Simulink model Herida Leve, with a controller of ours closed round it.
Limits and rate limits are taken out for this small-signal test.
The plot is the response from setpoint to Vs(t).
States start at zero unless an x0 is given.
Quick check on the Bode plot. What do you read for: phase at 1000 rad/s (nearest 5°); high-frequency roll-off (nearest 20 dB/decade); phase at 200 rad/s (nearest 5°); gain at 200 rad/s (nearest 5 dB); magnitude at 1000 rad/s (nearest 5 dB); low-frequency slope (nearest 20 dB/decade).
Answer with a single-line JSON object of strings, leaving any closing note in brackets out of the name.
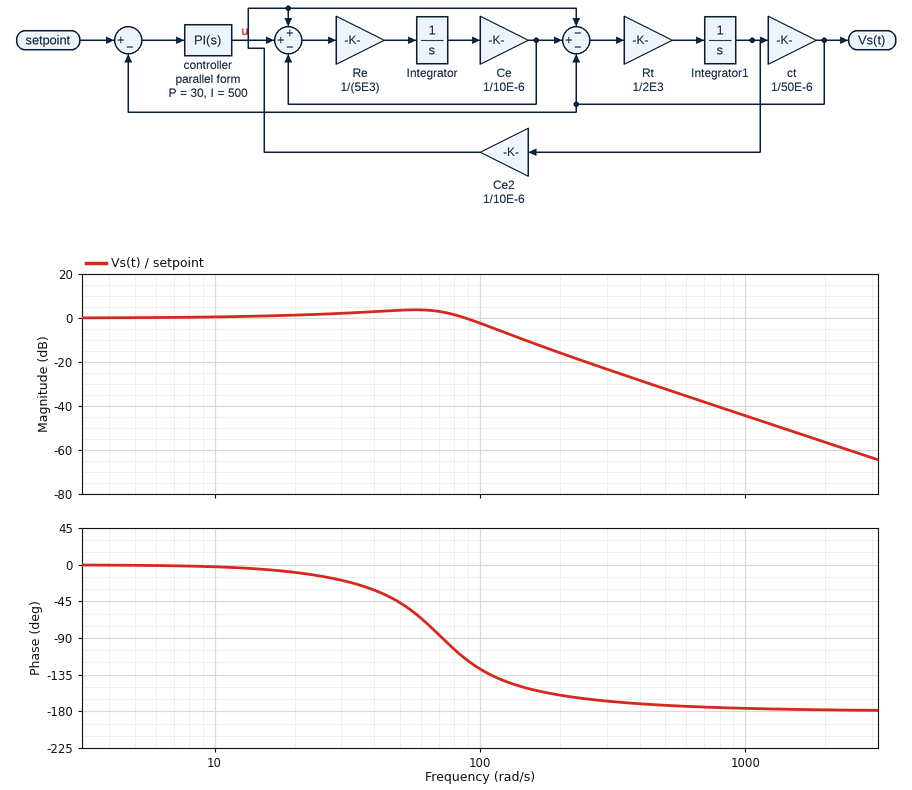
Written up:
{"phase at 1000 rad/s": "-175°", "high-frequency roll-off": "-40 dB/decade", "phase at 200 rad/s": "-160°", "gain at 200 rad/s": "-15 dB", "magnitude at 1000 rad/s": "-45 dB", "low-frequency slope": "0 dB/decade"}
